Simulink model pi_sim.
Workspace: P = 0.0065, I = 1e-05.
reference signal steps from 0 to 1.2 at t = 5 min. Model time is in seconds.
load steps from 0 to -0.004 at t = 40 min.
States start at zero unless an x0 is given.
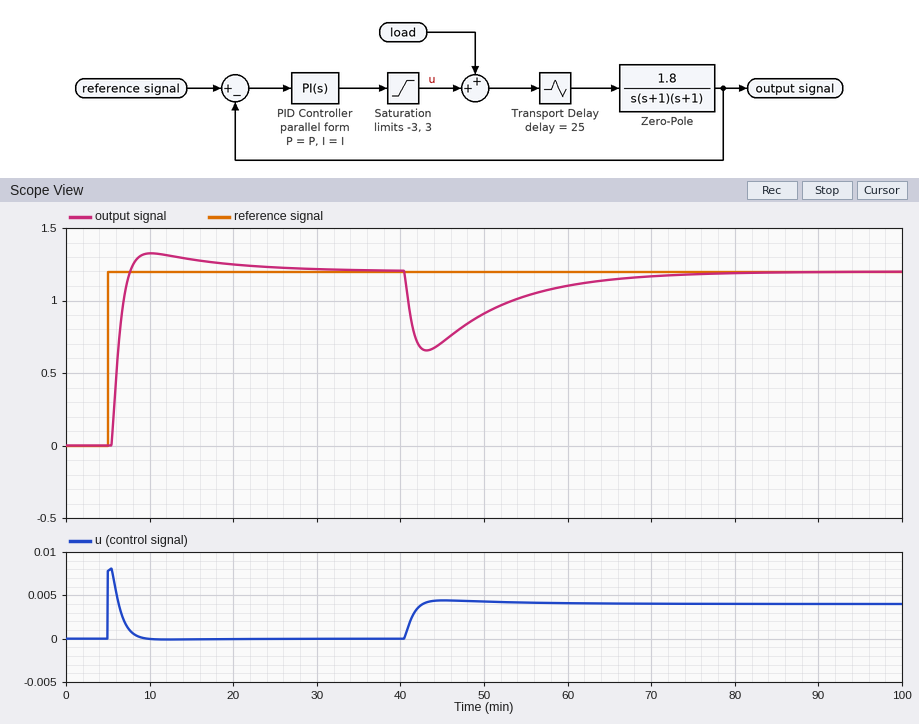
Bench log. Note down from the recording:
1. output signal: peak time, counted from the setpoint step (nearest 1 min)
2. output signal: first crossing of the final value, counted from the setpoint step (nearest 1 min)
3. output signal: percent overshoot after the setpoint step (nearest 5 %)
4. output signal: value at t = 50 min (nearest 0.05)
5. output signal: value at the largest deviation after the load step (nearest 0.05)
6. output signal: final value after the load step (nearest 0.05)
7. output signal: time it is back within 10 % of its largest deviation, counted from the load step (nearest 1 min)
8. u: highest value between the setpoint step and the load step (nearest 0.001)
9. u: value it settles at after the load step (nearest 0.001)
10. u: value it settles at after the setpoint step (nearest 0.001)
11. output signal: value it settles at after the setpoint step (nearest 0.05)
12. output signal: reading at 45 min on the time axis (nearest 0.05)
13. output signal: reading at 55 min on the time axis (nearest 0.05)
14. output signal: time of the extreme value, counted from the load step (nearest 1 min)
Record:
5 min
3 min
10 %
0.90
0.65
1.20
25 min
0.008
0.004
0.000
1.20
0.70
1.05
3 min
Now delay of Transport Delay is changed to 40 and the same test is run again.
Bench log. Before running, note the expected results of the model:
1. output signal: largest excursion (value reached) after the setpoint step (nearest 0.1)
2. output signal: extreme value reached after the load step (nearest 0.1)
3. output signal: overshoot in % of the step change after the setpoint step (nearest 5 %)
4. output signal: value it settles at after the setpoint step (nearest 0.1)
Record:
1.4
0.6
15 %
1.2
